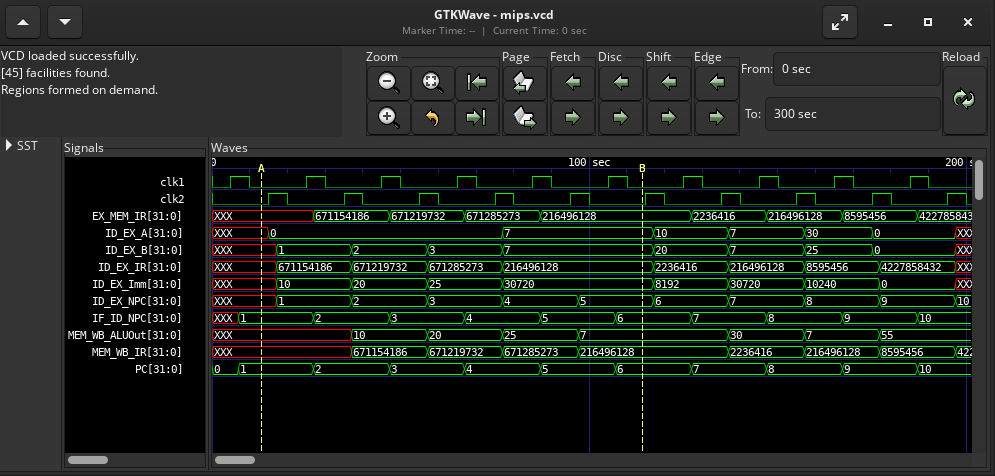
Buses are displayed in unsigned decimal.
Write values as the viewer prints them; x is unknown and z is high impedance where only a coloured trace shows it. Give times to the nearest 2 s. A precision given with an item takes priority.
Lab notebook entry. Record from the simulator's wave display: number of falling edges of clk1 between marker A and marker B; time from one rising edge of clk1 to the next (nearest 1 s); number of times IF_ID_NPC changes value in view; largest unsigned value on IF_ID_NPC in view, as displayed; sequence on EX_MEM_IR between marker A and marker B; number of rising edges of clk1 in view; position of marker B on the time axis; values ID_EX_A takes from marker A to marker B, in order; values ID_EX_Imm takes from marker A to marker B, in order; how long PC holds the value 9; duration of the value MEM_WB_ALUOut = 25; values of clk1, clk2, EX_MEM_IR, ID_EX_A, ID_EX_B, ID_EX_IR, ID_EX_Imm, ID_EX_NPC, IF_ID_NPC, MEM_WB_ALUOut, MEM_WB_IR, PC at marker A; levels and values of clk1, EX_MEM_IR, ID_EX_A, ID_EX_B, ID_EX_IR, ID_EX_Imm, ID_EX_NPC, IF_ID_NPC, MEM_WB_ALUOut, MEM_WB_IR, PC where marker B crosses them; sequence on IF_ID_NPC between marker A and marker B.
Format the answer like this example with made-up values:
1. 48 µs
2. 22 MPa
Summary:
1. 5
2. 20 s
3. 10
4. 10
5. XXX, 671154186, 671219732, 671285273, 216496128
6. 10
7. 114 s
8. XXX, 0, 7
9. XXX, 10, 20, 25, 30720
10. 20 s
11. 20 s
12. clk1=0, clk2=0, EX_MEM_IR=XXX, ID_EX_A=XXX, ID_EX_B=XXX, ID_EX_IR=XXX, ID_EX_Imm=XXX, ID_EX_NPC=XXX, IF_ID_NPC=1, MEM_WB_ALUOut=XXX, MEM_WB_IR=XXX, PC=1
13. clk1=0, EX_MEM_IR=216496128, ID_EX_A=7, ID_EX_B=7, ID_EX_IR=216496128, ID_EX_Imm=30720, ID_EX_NPC=5, IF_ID_NPC=6, MEM_WB_ALUOut=7, MEM_WB_IR=216496128, PC=6
14. 1, 2, 3, 4, 5, 6
